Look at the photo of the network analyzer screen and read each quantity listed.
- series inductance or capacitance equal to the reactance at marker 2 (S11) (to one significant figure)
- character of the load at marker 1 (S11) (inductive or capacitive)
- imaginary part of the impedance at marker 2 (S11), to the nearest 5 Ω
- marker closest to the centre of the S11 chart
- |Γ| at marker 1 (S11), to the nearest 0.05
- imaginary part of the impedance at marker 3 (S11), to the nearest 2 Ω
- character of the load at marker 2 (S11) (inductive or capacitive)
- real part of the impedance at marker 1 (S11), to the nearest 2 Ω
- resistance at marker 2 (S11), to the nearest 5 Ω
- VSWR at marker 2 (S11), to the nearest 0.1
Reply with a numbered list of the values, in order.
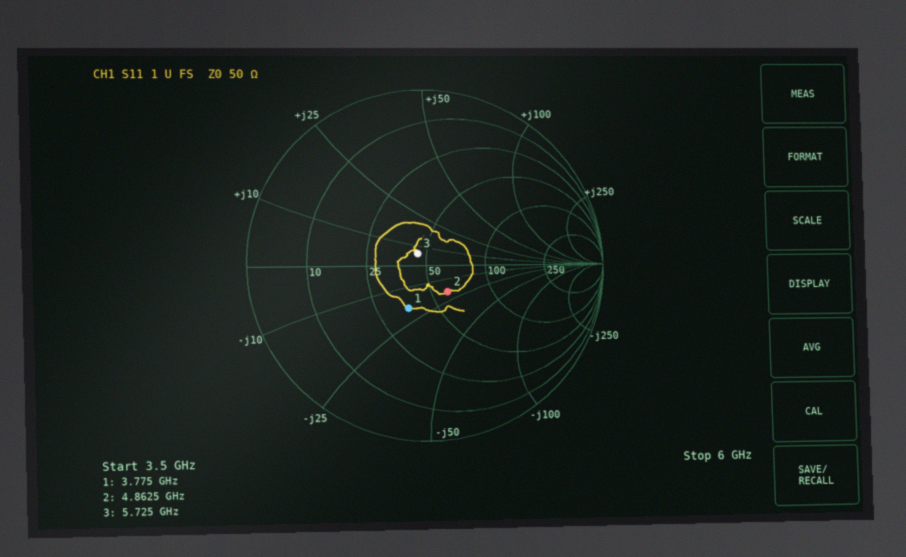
1. 2 pF
2. capacitive
3. -20 Ω
4. marker 3
5. 0.25
6. +6 Ω
7. capacitive
8. 36 Ω
9. 60 Ω
10. 1.5
